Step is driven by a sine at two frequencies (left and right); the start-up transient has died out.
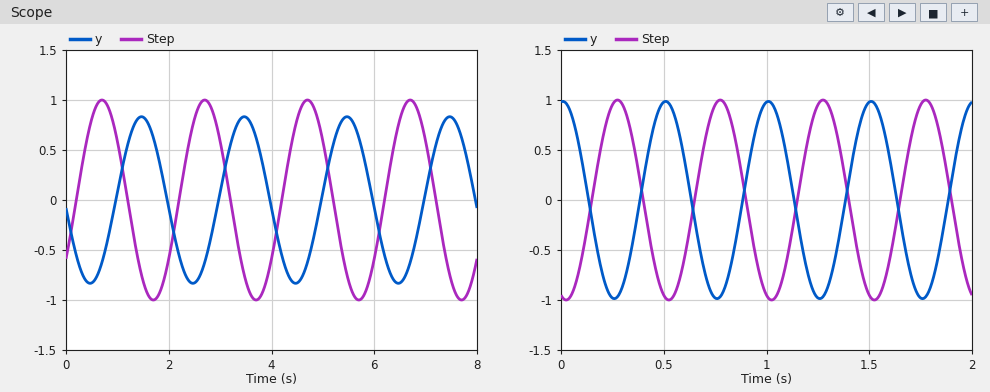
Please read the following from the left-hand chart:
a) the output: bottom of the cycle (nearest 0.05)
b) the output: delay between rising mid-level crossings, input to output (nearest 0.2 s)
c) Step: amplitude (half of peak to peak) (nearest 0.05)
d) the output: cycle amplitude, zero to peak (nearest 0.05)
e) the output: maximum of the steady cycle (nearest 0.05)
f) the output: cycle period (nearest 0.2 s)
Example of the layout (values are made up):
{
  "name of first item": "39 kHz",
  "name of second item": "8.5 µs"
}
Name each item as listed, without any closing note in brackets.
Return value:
{
  "the output: bottom of the cycle": "-0.85",
  "the output: delay between rising mid-level crossings, input to output": "0.8 s",
  "Step: amplitude (half of peak to peak)": "1.00",
  "the output: cycle amplitude, zero to peak": "0.85",
  "the output: maximum of the steady cycle": "0.85",
  "the output: cycle period": "2.0 s"
}
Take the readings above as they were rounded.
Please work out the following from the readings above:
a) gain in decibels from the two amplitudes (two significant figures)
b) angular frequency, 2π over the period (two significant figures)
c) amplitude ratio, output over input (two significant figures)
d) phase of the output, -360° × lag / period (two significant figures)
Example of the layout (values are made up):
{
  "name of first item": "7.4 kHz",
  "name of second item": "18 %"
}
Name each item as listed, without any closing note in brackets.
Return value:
{
  "gain in decibels from the two amplitudes": "-1.4 dB",
  "angular frequency, 2π over the period": "3.1 rad/s",
  "amplitude ratio, output over input": "0.85",
  "phase of the output, -360° × lag / period": "-140°"
}
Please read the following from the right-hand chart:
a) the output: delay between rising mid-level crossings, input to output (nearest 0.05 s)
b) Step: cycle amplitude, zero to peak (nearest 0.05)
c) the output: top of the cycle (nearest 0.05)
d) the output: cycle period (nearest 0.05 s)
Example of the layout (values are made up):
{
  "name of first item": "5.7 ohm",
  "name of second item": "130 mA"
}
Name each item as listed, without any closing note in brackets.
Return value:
{
  "the output: delay between rising mid-level crossings, input to output": "0.25 s",
  "Step: cycle amplitude, zero to peak": "1.00",
  "the output: top of the cycle": "1.00",
  "the output: cycle period": "0.50 s"
}
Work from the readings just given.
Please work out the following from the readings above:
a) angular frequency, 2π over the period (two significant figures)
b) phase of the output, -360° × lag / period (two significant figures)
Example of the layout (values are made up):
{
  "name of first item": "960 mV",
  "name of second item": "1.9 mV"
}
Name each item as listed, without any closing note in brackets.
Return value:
{
  "angular frequency, 2π over the period": "13 rad/s",
  "phase of the output, -360° × lag / period": "-180°"
}
